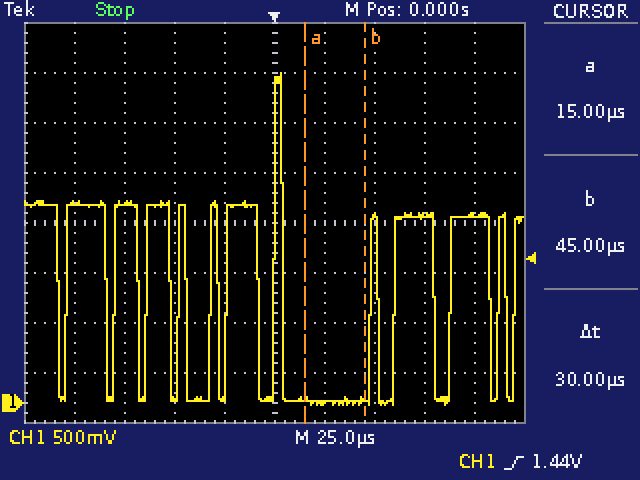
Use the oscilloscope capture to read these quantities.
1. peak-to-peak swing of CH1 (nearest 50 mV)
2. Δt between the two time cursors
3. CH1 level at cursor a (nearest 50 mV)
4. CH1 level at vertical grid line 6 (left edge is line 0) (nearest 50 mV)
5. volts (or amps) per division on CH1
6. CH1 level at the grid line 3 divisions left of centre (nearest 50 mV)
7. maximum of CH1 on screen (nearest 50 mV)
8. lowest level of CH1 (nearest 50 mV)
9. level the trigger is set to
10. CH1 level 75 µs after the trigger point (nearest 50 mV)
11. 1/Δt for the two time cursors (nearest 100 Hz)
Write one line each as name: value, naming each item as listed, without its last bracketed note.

peak-to-peak swing of CH1: 3.30 V
Δt between the two time cursors: 30 µs
CH1 level at cursor a: 0 mV
CH1 level at vertical grid line 6 (left edge is line 0): 0 mV
volts (or amps) per division on CH1: 500 mV
CH1 level at the grid line 3 divisions left of centre: 2.00 V
maximum of CH1 on screen: 3.30 V
lowest level of CH1: 0 mV
level the trigger is set to: 1.44 V
CH1 level 75 µs after the trigger point: 1.85 V
1/Δt for the two time cursors: 33.3 kHz
